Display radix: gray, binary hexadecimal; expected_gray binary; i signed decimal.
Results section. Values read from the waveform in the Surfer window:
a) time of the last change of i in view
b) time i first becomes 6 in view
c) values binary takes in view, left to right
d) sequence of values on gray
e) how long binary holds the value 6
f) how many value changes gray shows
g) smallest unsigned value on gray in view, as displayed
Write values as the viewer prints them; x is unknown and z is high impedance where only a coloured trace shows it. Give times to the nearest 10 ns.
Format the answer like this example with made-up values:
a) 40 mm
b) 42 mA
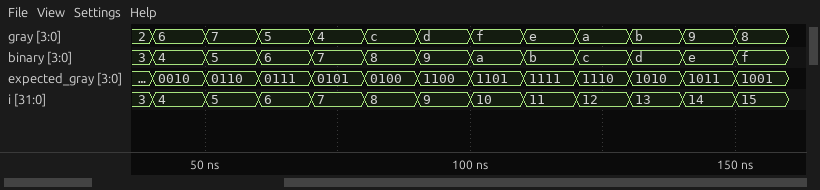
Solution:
a) 150 ns
b) 60 ns
c) 3, 4, 5, 6, 7, 8, 9, a, b, c, d, e, f
d) 2, 6, 7, 5, 4, c, d, f, e, a, b, 9, 8
e) 10 ns
f) 12
g) 2
